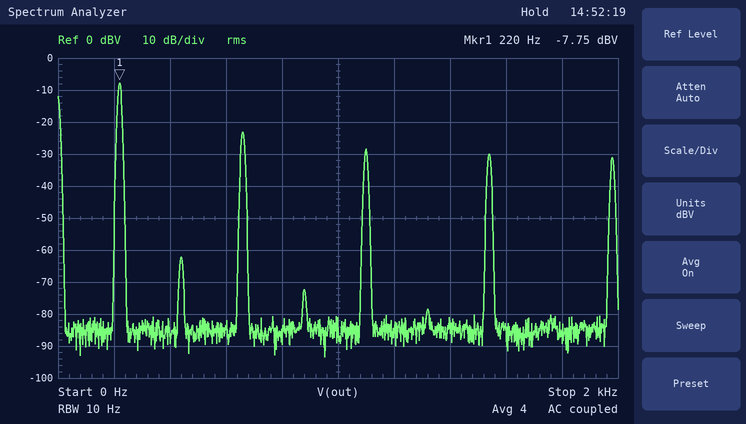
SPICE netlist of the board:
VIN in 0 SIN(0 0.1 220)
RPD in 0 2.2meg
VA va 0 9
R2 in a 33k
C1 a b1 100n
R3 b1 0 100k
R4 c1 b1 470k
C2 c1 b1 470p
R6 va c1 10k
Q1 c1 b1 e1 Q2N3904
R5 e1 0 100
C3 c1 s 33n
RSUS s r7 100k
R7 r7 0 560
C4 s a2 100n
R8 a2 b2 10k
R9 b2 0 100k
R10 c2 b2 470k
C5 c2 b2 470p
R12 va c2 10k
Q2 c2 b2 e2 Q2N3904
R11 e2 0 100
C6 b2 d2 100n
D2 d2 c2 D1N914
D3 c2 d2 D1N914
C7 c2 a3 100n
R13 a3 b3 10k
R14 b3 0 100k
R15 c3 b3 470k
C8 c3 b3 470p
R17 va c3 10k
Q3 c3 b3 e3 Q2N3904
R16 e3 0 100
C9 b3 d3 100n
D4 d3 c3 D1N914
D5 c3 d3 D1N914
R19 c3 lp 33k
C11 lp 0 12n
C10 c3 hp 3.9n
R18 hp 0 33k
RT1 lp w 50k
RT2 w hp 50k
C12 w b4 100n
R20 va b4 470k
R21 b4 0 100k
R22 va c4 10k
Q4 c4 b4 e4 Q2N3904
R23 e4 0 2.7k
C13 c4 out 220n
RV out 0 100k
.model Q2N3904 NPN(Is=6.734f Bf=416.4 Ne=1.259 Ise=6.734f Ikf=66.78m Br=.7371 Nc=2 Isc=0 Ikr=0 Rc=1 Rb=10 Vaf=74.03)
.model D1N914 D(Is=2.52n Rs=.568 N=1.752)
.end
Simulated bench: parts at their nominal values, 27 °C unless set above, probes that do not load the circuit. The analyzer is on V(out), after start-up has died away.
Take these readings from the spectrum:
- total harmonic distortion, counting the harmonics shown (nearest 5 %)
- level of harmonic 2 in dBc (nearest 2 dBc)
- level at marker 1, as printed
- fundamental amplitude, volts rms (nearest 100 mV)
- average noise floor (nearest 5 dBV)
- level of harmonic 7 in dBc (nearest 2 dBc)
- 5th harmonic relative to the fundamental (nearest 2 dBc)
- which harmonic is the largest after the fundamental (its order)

20 %
-54 dBc
-7.75 dBV
400 mV
-85 dBV
-22 dBc
-20 dBc
3
